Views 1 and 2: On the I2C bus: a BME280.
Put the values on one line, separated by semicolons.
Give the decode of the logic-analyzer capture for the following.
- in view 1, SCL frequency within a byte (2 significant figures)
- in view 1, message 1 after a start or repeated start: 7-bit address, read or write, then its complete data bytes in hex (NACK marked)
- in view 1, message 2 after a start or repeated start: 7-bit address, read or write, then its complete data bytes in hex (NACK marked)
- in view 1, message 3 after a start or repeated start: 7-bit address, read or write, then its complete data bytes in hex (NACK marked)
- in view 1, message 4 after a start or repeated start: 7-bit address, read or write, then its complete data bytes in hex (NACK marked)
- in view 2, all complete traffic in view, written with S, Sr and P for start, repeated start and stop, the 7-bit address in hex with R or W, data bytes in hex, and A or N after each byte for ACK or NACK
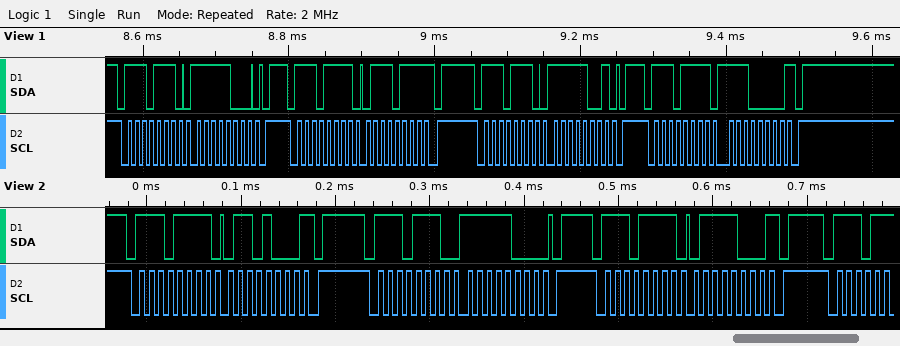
100 kHz; 0x77 write: F8; 0x77 read: 77 NACK; 0x77 write: F9; 0x77 read: E0 NACK; S 77R A 68 N P S 77W A F8 A P S 77R A 78 N P
